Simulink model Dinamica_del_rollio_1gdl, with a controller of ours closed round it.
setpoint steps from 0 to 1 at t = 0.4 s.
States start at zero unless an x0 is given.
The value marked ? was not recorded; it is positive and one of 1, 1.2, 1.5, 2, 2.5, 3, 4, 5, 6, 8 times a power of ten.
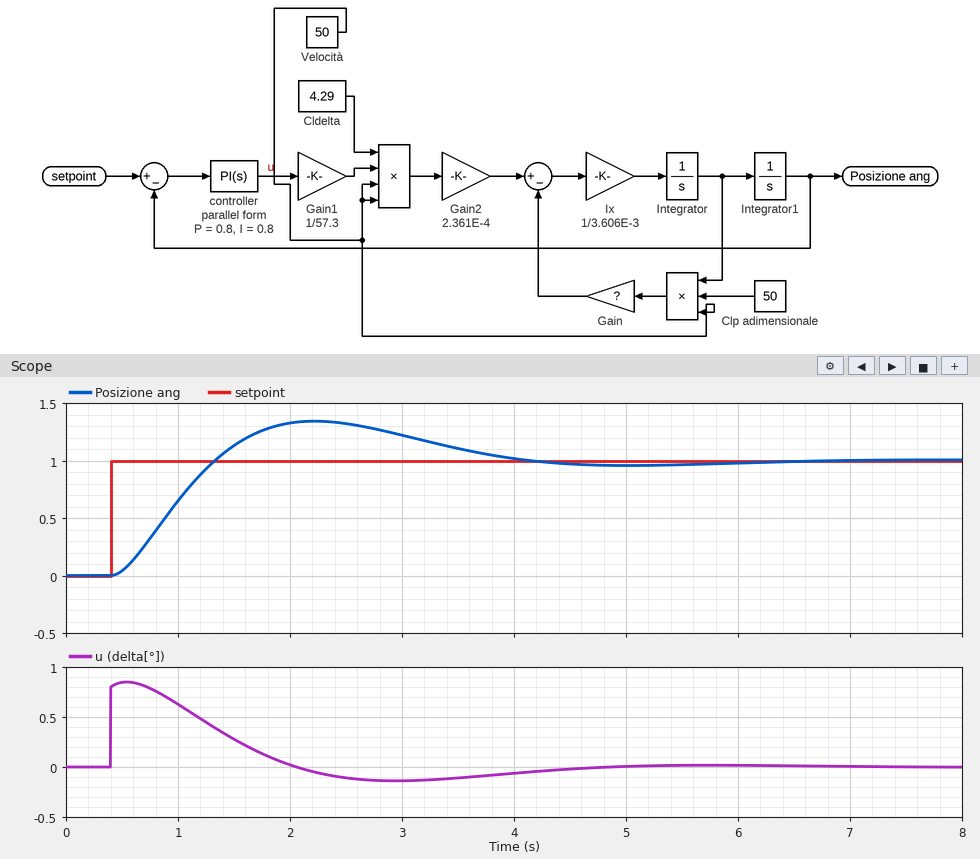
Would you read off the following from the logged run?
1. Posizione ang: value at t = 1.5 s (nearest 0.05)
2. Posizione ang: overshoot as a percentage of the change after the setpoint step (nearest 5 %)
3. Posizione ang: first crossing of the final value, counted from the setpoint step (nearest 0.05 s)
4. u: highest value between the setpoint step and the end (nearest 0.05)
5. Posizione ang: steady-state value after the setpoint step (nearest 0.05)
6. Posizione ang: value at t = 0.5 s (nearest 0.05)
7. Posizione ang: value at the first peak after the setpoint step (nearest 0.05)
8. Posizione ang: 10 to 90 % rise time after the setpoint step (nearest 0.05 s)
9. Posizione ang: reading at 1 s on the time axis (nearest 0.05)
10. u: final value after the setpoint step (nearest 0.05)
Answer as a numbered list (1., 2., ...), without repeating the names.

1. 1.15
2. 35 %
3. 0.95 s
4. 0.85
5. 1.00
6. 0.05
7. 1.35
8. 0.65 s
9. 0.65
10. 0.00
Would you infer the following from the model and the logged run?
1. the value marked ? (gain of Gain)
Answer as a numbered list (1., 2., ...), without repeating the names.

1. 1e-05
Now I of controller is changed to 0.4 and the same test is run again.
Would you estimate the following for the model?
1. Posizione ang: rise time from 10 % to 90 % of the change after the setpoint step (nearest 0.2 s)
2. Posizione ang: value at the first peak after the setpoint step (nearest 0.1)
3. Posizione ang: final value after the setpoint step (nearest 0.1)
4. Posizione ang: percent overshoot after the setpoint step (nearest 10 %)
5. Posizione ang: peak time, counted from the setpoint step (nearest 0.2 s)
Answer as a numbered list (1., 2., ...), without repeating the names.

1. 0.8 s
2. 1.2
3. 1.0
4. 20 %
5. 2.2 s
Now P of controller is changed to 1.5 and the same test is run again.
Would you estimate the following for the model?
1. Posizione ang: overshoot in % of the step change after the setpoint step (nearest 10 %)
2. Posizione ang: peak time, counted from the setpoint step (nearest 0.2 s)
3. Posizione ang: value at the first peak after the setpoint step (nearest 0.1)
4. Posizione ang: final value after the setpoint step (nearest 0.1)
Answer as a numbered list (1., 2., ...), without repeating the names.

1. 20 %
2. 1.2 s
3. 1.2
4. 1.0
